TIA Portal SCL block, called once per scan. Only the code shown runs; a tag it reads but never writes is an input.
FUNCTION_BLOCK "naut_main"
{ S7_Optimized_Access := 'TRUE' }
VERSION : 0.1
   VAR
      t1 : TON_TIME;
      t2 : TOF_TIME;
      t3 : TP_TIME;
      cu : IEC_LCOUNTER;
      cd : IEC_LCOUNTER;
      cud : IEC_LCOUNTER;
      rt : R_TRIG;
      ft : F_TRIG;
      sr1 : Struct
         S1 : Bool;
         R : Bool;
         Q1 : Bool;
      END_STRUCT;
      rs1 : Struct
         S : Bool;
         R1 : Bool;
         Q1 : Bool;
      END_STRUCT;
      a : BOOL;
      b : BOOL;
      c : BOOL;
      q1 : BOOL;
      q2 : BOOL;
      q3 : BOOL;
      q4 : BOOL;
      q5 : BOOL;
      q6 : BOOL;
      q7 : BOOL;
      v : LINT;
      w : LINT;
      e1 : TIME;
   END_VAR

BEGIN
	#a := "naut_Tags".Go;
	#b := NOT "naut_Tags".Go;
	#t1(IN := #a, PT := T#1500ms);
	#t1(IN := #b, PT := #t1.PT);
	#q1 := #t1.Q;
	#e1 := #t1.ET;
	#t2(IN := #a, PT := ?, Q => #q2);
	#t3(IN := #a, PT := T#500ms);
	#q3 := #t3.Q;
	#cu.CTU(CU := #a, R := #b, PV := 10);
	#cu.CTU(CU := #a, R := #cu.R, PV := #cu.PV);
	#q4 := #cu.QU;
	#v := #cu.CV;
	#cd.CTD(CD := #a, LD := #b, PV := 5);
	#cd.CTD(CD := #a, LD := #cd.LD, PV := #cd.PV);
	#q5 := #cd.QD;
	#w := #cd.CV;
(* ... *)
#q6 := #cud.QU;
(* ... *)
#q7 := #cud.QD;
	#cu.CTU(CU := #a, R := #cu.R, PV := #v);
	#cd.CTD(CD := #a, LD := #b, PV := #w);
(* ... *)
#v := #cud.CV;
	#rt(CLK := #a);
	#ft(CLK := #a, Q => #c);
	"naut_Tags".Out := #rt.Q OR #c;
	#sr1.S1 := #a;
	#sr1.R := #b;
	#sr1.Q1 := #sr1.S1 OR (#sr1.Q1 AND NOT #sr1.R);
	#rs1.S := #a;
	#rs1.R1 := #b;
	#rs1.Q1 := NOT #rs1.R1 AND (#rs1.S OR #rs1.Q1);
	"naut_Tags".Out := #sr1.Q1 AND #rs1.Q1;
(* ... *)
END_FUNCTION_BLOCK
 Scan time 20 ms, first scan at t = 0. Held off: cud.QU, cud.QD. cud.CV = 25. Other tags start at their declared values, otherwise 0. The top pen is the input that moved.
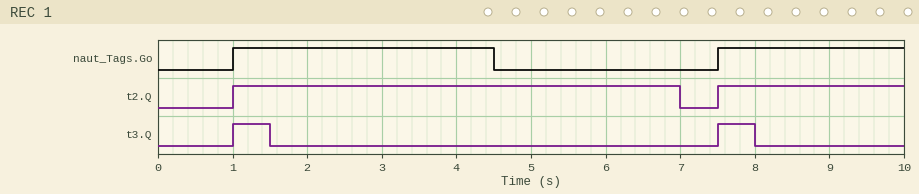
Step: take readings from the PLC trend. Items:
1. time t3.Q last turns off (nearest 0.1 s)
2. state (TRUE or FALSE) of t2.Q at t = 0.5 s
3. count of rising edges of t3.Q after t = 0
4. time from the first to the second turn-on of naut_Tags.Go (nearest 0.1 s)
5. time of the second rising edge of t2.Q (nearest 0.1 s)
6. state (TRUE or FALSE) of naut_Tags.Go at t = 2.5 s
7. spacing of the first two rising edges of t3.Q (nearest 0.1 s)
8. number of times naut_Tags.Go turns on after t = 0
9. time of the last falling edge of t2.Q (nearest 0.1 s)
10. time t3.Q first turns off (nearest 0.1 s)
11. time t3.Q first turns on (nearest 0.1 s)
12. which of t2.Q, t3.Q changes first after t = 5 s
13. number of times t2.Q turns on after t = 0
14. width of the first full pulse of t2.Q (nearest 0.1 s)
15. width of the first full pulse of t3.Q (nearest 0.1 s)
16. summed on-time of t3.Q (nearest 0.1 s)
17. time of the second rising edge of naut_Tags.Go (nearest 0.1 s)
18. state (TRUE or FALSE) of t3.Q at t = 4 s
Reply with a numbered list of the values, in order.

1. 8.0 s
2. FALSE
3. 2
4. 6.5 s
5. 7.5 s
6. TRUE
7. 6.5 s
8. 2
9. 7.0 s
10. 1.5 s
11. 1.0 s
12. t2.Q
13. 2
14. 6.0 s
15. 0.5 s
16. 1.0 s
17. 7.5 s
18. FALSE
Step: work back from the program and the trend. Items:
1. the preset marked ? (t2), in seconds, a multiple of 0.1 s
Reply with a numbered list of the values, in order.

1. 2.5 s
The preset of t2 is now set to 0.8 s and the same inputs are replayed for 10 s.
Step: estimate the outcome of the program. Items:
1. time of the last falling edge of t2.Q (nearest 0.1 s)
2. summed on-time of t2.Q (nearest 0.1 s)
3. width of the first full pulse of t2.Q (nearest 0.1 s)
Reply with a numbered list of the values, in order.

1. 5.3 s
2. 6.8 s
3. 4.3 s
